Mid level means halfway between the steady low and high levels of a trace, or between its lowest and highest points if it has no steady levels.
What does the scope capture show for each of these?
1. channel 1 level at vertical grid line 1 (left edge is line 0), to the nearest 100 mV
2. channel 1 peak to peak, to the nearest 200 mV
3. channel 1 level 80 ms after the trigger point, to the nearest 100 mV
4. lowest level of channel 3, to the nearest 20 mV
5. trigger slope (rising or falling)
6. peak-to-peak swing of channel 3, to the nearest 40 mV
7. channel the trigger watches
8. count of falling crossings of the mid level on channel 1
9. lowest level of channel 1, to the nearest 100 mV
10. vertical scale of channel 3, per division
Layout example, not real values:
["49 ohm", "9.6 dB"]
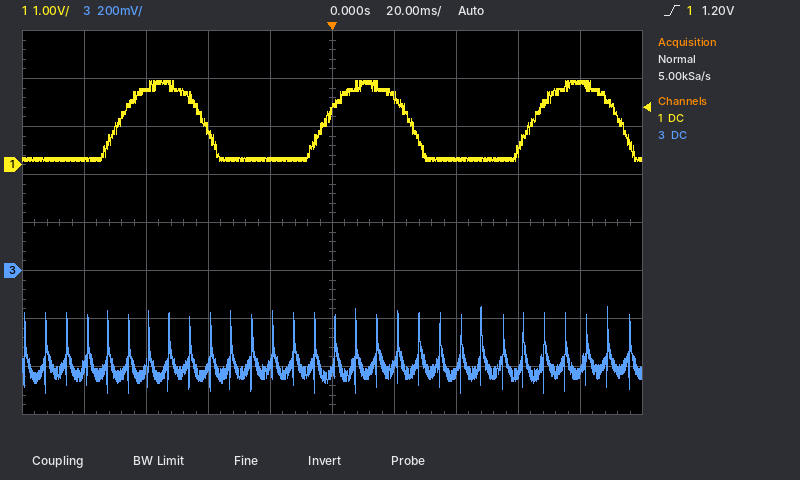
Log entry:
["100 mV", "1.6 V", "1.7 V", "-520 mV", "rising", "360 mV", "channel 1", "3", "100 mV", "200 mV"]
